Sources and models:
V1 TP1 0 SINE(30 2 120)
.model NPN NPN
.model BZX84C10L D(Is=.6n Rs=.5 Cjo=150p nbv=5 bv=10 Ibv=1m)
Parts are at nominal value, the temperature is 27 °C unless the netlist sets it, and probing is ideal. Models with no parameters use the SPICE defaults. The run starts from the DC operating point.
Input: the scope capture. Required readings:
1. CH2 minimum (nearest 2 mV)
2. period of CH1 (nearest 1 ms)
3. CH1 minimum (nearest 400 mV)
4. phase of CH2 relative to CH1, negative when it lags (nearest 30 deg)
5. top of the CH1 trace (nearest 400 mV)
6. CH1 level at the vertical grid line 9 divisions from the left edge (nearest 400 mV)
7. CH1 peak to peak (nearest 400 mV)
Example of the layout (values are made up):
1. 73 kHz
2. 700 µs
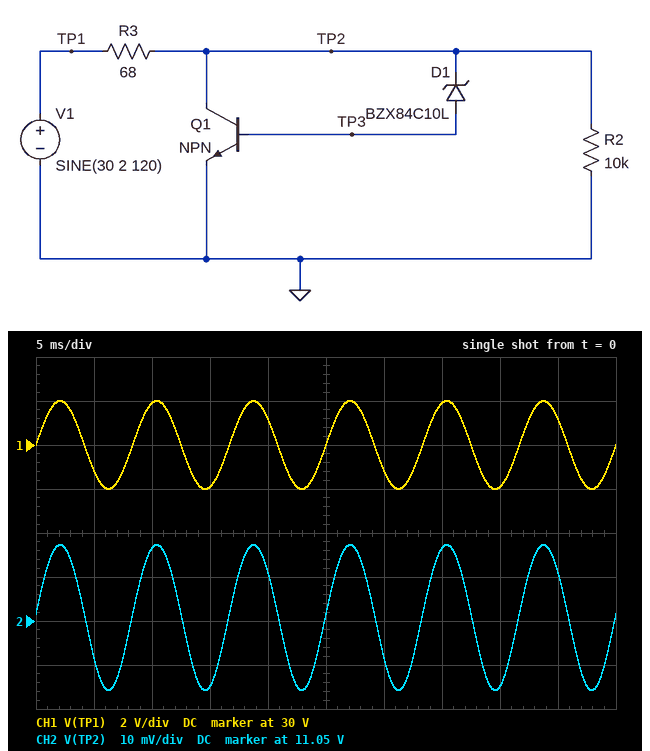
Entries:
1. 11.034 V
2. 8 ms
3. 28.0 V
4. 0 deg
5. 32.0 V
6. 31.2 V
7. 4.0 V
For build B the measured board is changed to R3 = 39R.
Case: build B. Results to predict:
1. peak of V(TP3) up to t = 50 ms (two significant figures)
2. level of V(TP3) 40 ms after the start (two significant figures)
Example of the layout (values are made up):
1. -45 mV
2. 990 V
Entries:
1. 940 mV
2. 930 mV
